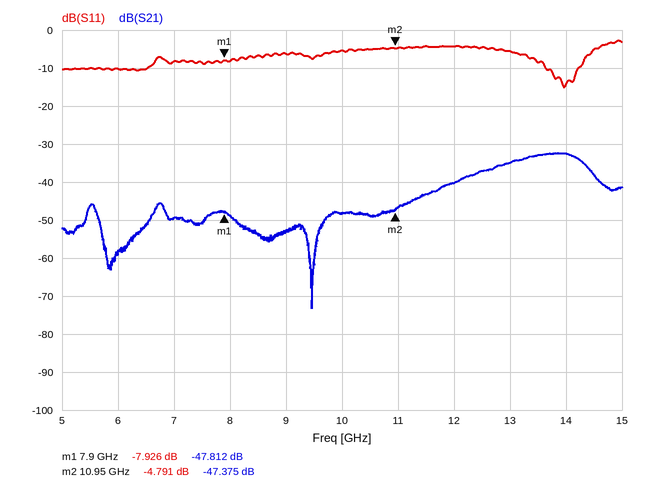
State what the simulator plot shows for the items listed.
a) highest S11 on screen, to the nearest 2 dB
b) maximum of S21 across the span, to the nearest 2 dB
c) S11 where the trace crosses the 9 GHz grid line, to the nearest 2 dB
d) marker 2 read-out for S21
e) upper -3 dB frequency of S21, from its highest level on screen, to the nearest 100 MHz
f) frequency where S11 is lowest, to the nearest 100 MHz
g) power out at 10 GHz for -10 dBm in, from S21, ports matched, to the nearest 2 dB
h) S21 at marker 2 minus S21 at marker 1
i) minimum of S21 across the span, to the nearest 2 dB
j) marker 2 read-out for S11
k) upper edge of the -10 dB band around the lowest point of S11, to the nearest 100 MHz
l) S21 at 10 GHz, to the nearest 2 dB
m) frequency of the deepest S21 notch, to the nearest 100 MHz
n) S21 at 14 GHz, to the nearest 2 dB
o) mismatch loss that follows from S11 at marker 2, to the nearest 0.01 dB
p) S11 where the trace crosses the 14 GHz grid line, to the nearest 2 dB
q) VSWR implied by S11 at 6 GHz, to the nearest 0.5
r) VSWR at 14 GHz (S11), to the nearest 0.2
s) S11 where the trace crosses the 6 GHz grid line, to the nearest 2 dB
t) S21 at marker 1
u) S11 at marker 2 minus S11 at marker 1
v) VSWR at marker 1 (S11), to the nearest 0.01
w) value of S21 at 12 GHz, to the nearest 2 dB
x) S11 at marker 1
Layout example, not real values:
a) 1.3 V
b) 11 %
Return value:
a) -2 dB
b) -32 dB
c) -6 dB
d) -47.375 dB
e) 14.3 GHz
f) 14.0 GHz
g) -58 dBm
h) 0.437 dB
i) -74 dB
j) -4.791 dB
k) 14.2 GHz
l) -48 dB
m) 9.5 GHz
n) -32 dB
o) 1.75 dB
p) -14 dB
q) 2.0
r) 1.4
s) -10 dB
t) -47.812 dB
u) 3.135 dB
v) 2.34
w) -40 dB
x) -7.926 dB
